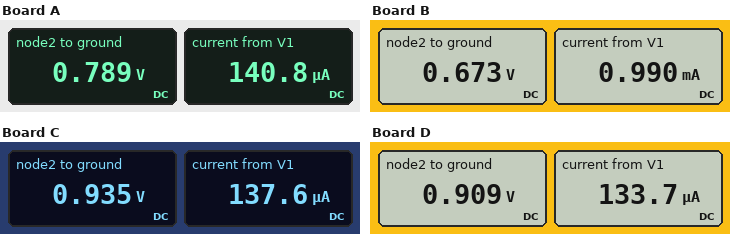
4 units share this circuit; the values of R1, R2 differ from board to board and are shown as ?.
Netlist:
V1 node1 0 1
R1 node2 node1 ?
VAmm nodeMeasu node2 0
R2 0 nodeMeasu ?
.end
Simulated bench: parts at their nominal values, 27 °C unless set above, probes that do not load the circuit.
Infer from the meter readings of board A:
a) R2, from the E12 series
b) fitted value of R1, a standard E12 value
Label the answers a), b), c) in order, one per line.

a) 5.6 kΩ
b) 1.5 kΩ
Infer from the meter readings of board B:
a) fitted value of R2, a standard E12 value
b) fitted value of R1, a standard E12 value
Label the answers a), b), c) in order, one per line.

a) 680 Ω
b) 330 Ω
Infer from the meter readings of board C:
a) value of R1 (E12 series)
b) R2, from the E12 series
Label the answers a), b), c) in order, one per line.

a) 470 Ω
b) 6.8 kΩ
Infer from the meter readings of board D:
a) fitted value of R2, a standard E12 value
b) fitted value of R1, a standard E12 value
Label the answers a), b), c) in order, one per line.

a) 6.8 kΩ
b) 680 Ω
